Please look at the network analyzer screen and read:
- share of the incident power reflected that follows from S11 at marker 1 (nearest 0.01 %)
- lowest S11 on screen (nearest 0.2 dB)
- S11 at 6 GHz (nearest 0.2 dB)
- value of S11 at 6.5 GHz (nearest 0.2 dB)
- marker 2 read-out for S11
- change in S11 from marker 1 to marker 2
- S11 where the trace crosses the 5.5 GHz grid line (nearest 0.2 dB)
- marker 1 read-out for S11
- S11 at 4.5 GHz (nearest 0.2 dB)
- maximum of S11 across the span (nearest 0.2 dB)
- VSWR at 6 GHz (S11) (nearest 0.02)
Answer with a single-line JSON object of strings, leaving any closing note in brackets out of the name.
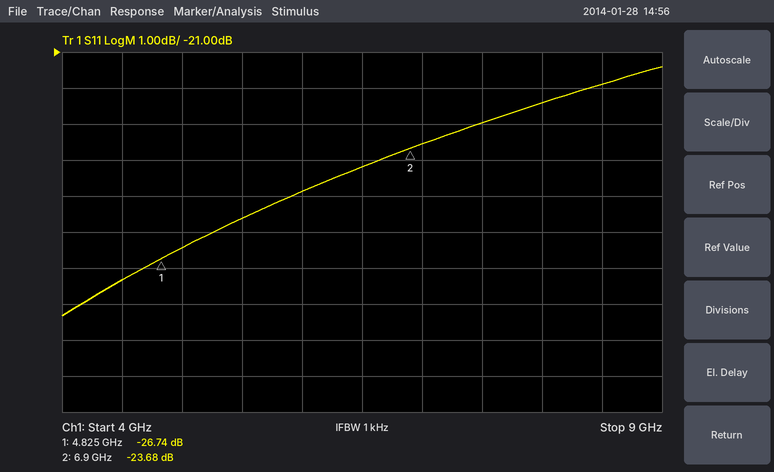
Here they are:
{"share of the incident power reflected that follows from S11 at marker 1": "0.21 %", "lowest S11 on screen": "-28.4 dB", "S11 at 6 GHz": "-24.8 dB", "value of S11 at 6.5 GHz": "-24.2 dB", "marker 2 read-out for S11": "-23.68 dB", "change in S11 from marker 1 to marker 2": "3.06 dB", "S11 where the trace crosses the 5.5 GHz grid line": "-25.6 dB", "marker 1 read-out for S11": "-26.74 dB", "S11 at 4.5 GHz": "-27.4 dB", "maximum of S11 across the span": "-21.4 dB", "VSWR at 6 GHz (S11)": "1.12"}
